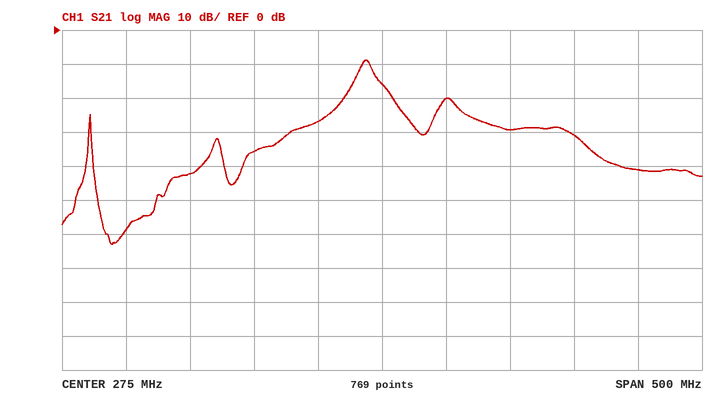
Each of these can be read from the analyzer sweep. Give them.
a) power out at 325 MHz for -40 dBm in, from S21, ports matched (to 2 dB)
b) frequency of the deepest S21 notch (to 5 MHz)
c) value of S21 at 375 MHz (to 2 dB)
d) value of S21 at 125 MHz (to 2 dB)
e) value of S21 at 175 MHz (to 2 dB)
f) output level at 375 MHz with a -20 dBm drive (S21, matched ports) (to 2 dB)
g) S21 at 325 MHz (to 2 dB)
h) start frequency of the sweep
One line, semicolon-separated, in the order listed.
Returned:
-60 dBm; 65 MHz; -30 dB; -42 dB; -36 dB; -50 dBm; -20 dB; 25 MHz
